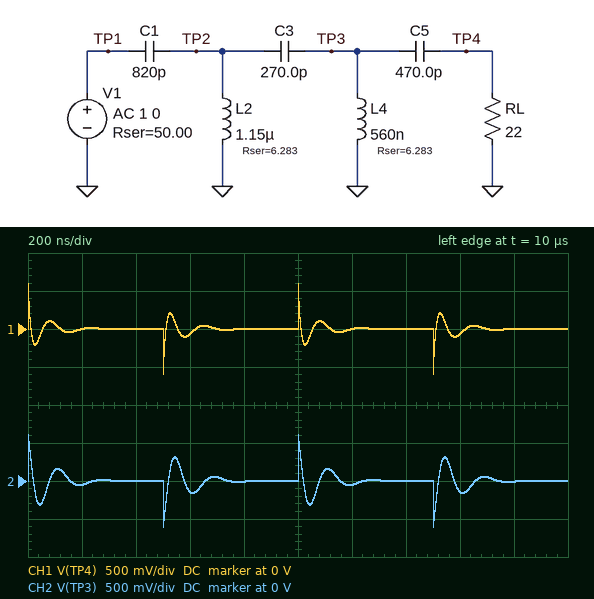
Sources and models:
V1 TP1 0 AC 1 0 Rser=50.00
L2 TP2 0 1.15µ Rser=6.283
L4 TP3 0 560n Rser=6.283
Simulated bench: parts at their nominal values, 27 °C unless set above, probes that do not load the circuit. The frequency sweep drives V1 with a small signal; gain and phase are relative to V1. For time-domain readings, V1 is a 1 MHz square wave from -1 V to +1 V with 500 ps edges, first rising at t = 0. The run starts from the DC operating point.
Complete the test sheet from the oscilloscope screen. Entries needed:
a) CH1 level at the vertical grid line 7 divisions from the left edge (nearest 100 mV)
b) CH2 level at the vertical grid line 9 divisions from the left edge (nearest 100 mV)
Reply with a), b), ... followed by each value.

a) 0 V
b) 0 V
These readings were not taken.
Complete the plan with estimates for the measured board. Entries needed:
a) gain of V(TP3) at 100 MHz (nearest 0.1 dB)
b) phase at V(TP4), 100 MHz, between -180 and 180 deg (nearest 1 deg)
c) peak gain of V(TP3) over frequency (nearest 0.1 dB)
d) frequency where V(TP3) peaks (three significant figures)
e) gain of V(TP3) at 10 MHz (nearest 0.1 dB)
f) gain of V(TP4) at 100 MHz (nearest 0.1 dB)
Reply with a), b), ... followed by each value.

a) -10.2 dB
b) 13 deg
c) -6.1 dB
d) 8.98 MHz
e) -6.2 dB
f) -10.3 dB
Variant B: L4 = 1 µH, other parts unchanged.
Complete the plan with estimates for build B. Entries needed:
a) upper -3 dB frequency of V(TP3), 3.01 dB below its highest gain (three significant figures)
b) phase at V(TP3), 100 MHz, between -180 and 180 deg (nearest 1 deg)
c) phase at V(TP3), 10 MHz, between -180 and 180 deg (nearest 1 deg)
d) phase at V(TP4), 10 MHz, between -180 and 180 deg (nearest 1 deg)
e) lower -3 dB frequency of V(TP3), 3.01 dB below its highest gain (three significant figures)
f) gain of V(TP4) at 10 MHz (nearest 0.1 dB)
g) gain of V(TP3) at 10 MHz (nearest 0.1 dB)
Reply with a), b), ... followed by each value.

a) 12.5 MHz
b) 3 deg
c) 53 deg
d) 110 deg
e) 4.92 MHz
f) -11.6 dB
g) -6.4 dB
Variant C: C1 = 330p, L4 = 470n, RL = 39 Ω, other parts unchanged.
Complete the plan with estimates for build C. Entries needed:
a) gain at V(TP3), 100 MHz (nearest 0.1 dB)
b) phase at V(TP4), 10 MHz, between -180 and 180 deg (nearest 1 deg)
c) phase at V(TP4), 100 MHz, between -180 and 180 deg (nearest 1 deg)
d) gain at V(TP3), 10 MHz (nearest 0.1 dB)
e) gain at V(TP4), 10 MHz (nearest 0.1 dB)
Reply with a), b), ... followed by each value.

a) -7.2 dB
b) 151 deg
c) 15 deg
d) -8.2 dB
e) -10.6 dB
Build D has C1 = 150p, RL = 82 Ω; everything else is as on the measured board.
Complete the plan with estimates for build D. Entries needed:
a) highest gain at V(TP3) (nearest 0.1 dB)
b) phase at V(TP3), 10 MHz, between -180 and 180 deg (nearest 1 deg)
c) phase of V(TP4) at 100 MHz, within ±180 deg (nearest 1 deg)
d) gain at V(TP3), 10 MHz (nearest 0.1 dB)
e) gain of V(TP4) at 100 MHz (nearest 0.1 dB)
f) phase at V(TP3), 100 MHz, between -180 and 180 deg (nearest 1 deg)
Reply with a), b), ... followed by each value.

a) -4.0 dB
b) 137 deg
c) 16 deg
d) -9.9 dB
e) -4.1 dB
f) 14 deg
